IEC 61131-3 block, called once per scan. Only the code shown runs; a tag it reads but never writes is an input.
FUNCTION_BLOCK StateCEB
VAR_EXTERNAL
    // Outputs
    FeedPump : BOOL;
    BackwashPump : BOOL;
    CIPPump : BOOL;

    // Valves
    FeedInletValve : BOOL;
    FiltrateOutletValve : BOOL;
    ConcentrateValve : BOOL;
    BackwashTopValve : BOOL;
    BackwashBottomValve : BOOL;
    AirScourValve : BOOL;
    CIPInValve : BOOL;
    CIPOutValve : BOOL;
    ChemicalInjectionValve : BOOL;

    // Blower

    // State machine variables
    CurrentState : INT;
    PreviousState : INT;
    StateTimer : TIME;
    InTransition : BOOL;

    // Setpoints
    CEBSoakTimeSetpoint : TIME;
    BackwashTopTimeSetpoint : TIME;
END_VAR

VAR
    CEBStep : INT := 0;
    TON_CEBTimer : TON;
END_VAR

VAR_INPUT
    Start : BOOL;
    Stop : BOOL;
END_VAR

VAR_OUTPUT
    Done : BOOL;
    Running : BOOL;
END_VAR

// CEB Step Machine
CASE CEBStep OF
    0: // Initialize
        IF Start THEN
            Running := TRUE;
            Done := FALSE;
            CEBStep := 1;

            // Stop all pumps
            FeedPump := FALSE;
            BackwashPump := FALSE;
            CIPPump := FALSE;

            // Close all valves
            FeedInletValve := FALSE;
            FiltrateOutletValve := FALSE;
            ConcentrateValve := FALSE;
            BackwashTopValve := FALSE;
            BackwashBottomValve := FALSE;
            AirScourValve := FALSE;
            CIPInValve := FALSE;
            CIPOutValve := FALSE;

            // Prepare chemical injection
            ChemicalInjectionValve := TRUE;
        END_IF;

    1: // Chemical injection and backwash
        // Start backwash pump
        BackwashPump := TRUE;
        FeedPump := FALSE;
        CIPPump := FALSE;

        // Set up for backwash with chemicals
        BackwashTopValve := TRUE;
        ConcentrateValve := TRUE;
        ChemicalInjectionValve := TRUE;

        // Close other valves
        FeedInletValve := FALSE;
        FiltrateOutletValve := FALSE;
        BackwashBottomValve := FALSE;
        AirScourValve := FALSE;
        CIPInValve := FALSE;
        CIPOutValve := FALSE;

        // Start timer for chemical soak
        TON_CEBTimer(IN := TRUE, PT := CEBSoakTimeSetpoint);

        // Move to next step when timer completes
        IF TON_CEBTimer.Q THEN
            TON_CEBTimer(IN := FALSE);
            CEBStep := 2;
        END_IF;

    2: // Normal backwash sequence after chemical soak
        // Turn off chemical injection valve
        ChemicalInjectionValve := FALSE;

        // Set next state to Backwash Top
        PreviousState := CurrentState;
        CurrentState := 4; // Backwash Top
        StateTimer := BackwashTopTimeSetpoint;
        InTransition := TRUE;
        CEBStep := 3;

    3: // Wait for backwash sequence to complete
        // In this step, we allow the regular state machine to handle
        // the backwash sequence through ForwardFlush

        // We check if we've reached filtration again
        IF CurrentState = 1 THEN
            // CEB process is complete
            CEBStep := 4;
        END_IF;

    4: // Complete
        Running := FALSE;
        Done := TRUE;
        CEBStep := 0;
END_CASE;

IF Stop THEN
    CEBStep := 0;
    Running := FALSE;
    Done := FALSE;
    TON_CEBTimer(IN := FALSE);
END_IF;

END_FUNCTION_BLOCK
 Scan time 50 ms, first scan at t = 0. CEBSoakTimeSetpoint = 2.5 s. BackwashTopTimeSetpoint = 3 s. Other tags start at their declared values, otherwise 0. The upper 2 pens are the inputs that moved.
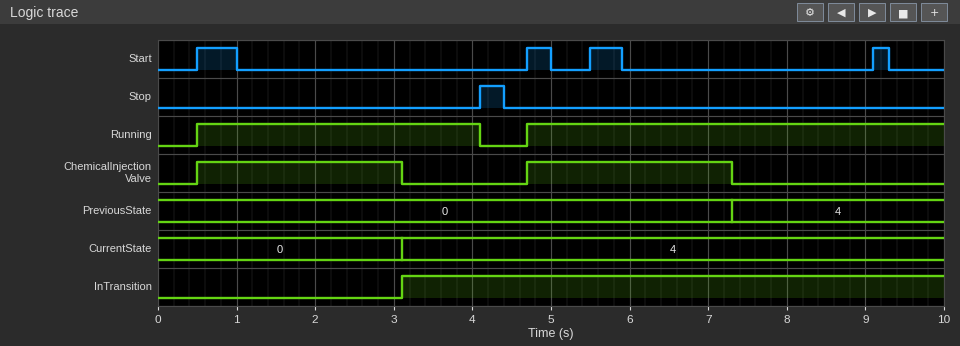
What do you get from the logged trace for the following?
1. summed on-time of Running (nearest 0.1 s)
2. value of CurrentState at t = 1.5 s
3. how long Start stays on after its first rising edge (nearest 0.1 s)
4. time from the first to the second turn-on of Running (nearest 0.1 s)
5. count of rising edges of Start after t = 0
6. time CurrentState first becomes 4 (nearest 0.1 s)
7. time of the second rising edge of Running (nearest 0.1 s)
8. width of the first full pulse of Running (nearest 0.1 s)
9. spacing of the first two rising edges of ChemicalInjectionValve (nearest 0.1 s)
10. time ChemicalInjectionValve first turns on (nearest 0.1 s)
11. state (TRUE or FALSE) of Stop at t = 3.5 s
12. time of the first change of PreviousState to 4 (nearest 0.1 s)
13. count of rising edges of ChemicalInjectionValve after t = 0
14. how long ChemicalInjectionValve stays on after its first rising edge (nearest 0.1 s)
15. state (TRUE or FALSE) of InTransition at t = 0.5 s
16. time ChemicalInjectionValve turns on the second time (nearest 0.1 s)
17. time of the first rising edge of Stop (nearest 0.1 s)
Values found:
8.9 s
0
0.5 s
4.2 s
4
3.1 s
4.7 s
3.6 s
4.2 s
0.5 s
FALSE
7.3 s
2
2.6 s
FALSE
4.7 s
4.1 s
